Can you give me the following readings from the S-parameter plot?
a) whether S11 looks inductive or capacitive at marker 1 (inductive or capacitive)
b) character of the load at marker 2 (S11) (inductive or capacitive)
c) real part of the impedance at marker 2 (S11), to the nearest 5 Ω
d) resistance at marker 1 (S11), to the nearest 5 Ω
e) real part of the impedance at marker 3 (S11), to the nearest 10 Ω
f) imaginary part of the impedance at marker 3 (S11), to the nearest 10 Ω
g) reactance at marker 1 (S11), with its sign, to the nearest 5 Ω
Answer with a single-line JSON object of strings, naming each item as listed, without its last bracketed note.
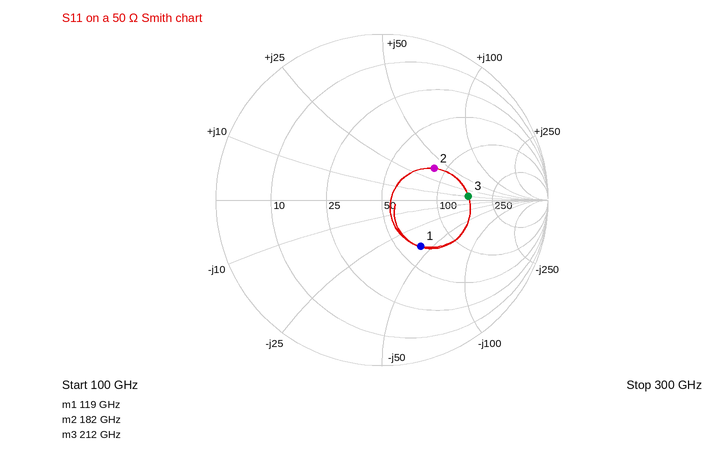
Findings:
{"whether S11 looks inductive or capacitive at marker 1": "capacitive", "character of the load at marker 2 (S11)": "inductive", "real part of the impedance at marker 2 (S11), to the nearest 5 Ω": "85 Ω", "resistance at marker 1 (S11), to the nearest 5 Ω": "65 Ω", "real part of the impedance at marker 3 (S11), to the nearest 10 Ω": "160 Ω", "imaginary part of the impedance at marker 3 (S11), to the nearest 10 Ω": "+10 Ω", "reactance at marker 1 (S11), with its sign, to the nearest 5 Ω": "-40 Ω"}
